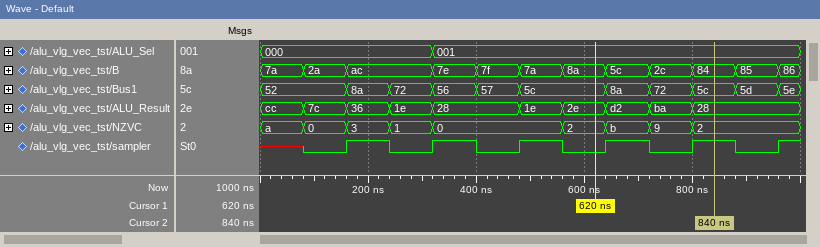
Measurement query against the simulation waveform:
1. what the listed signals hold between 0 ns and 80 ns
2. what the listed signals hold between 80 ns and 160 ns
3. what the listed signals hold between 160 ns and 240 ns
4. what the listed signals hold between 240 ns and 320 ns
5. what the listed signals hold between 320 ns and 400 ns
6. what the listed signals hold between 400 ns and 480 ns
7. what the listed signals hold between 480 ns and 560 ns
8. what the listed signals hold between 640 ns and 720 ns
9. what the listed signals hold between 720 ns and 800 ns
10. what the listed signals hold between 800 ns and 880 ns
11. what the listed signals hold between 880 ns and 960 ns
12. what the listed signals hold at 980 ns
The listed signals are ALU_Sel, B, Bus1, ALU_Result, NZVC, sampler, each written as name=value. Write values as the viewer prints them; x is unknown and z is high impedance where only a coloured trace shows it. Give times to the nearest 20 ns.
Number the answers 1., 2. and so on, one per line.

1. ALU_Sel=000, B=7a, Bus1=52, ALU_Result=cc, NZVC=a, sampler=x
2. ALU_Sel=000, B=2a, Bus1=52, ALU_Result=7c, NZVC=0, sampler=0
3. ALU_Sel=000, B=ac, Bus1=8a, ALU_Result=36, NZVC=3, sampler=1
4. ALU_Sel=000, B=ac, Bus1=72, ALU_Result=1e, NZVC=1, sampler=0
5. ALU_Sel=001, B=7e, Bus1=56, ALU_Result=28, NZVC=0, sampler=1
6. ALU_Sel=001, B=7f, Bus1=57, ALU_Result=28, NZVC=0, sampler=0
7. ALU_Sel=001, B=7a, Bus1=5c, ALU_Result=1e, NZVC=0, sampler=1
8. ALU_Sel=001, B=5c, Bus1=8a, ALU_Result=d2, NZVC=b, sampler=1
9. ALU_Sel=001, B=2c, Bus1=72, ALU_Result=ba, NZVC=9, sampler=0
10. ALU_Sel=001, B=84, Bus1=5c, ALU_Result=28, NZVC=2, sampler=1
11. ALU_Sel=001, B=85, Bus1=5d, ALU_Result=28, NZVC=2, sampler=0
12. ALU_Sel=001, B=86, Bus1=5e, ALU_Result=28, NZVC=2, sampler=1
